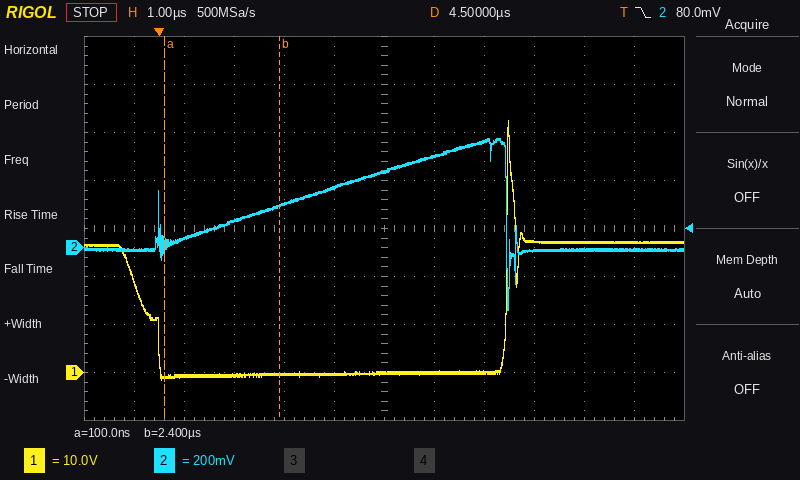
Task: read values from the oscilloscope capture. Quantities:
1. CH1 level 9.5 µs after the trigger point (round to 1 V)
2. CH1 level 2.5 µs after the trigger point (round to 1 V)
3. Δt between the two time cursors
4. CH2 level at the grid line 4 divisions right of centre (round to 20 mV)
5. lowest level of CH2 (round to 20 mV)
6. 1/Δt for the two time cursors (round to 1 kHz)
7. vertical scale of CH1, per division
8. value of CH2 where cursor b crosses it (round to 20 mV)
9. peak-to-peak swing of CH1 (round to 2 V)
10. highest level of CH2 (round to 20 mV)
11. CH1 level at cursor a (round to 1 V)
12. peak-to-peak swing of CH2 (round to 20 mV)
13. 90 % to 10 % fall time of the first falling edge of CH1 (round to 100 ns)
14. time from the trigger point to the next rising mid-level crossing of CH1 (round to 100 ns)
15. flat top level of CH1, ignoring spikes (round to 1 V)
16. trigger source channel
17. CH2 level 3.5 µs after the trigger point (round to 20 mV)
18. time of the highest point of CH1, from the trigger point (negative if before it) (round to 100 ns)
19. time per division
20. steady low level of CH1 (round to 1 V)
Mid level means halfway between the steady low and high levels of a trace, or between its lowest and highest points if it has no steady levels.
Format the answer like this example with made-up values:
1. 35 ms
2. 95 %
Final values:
1. 27 V
2. 0 V
3. 2.3 µs
4. 0 mV
5. -260 mV
6. 435 kHz
7. 10 V
8. 180 mV
9. 54 V
10. 460 mV
11. -1 V
12. 720 mV
13. 700 ns
14. 6.9 µs
15. 27 V
16. CH2
17. 260 mV
18. +7.0 µs
19. 1 µs
20. 0 V
